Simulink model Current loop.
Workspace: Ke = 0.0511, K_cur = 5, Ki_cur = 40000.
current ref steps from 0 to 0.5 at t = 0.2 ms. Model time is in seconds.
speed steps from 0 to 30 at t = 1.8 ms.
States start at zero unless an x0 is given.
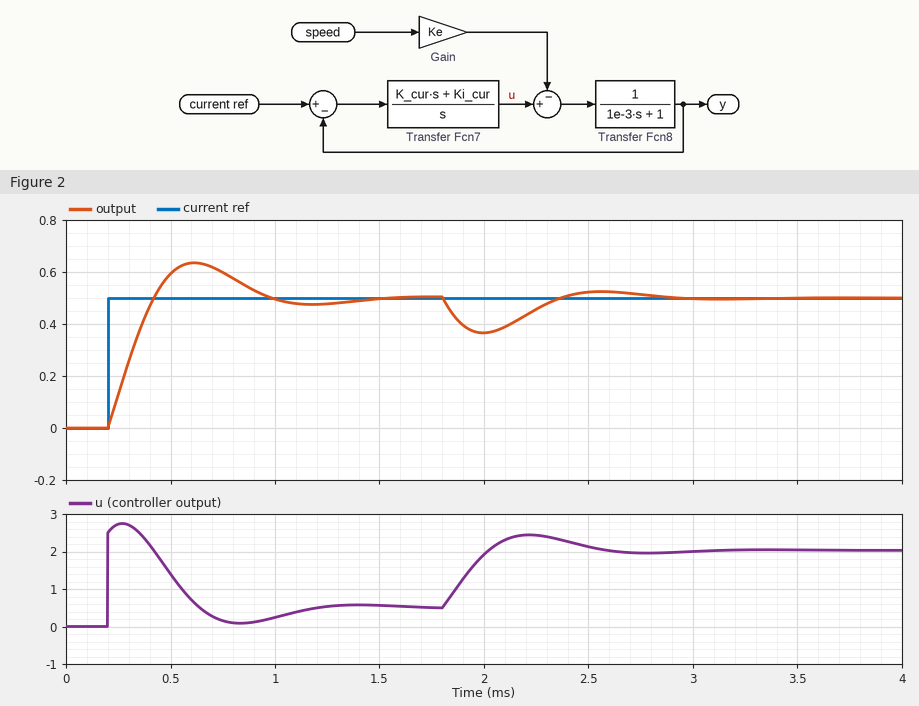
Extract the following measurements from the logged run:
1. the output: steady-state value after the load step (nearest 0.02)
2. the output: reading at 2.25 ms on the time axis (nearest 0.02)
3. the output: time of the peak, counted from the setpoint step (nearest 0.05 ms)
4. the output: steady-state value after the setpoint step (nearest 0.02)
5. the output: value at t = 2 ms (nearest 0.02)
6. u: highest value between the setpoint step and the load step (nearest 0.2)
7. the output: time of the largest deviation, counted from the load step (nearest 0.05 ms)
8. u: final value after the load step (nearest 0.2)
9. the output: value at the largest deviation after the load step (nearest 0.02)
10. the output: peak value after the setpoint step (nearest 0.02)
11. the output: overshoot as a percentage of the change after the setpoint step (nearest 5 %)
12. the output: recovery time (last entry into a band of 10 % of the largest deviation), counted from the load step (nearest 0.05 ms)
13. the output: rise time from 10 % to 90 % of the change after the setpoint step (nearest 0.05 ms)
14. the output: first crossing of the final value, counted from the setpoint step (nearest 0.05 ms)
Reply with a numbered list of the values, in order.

1. 0.50
2. 0.46
3. 0.40 ms
4. 0.50
5. 0.36
6. 2.8
7. 0.20 ms
8. 2.0
9. 0.36
10. 0.64
11. 25 %
12. 0.95 ms
13. 0.15 ms
14. 0.20 ms
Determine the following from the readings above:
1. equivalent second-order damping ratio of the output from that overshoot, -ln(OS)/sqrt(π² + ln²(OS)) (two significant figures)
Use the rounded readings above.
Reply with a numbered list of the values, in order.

1. 0.40
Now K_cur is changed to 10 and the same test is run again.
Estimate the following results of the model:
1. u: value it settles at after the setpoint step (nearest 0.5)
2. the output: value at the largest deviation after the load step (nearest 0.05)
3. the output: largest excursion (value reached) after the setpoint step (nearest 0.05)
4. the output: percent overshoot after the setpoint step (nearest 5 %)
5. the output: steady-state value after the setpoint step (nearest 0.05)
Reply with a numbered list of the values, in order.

1. 0.5
2. 0.40
3. 0.55
4. 10 %
5. 0.50
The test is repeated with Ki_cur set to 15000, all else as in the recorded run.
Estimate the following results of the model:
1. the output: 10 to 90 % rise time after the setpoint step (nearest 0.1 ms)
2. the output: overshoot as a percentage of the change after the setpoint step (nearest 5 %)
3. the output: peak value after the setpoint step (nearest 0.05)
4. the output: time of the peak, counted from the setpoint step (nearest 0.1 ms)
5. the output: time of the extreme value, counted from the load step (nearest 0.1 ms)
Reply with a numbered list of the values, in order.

1. 0.3 ms
2. 10 %
3. 0.55
4. 0.6 ms
5. 0.3 ms
